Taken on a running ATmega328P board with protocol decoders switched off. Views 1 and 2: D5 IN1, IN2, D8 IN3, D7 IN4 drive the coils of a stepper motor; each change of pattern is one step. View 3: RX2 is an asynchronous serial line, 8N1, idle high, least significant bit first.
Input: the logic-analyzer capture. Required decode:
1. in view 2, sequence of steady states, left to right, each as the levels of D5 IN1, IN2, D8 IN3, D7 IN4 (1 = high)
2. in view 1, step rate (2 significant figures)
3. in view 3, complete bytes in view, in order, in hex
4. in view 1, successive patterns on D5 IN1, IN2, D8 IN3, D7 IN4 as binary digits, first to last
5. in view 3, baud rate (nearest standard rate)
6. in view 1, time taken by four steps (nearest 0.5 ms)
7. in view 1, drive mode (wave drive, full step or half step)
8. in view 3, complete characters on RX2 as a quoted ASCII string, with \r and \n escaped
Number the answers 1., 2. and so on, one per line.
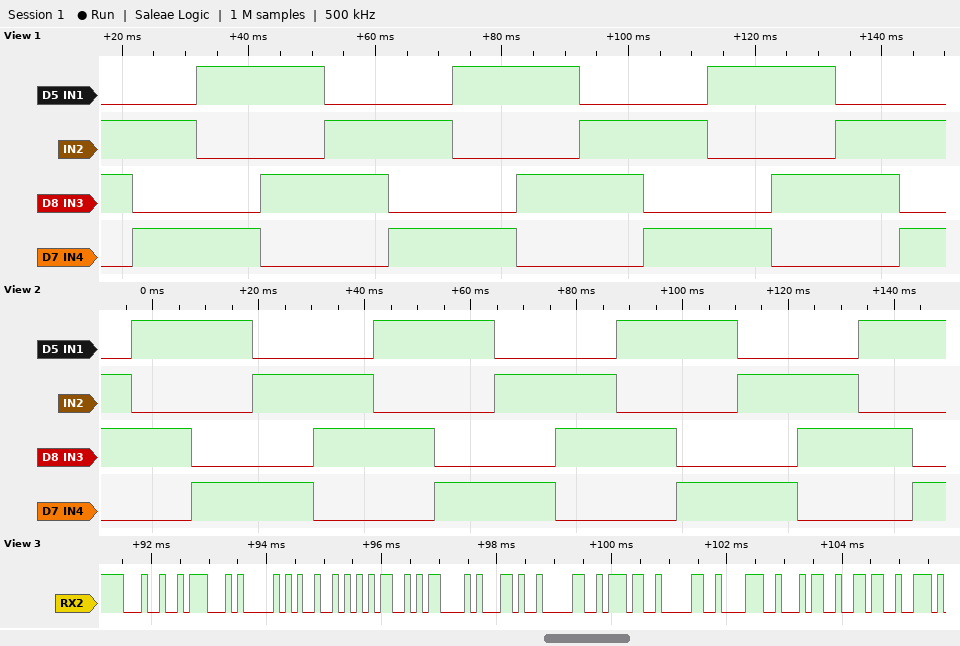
1. 0110 1010 1001 0101 0110 1010 1001 0101 0110 1010 1001 0101 0110 1010 1001
2. 99 steps/s
3. 24 47 50 52 4D 43 2C 30 37 30 38 34 36
4. 0110 0101 1001 1010 0110 0101 1001 1010 0110 0101 1001 1010 0110 0101
5. 9600 baud
6. 40.5 ms
7. full step
8. "$GPRMC,070846"
